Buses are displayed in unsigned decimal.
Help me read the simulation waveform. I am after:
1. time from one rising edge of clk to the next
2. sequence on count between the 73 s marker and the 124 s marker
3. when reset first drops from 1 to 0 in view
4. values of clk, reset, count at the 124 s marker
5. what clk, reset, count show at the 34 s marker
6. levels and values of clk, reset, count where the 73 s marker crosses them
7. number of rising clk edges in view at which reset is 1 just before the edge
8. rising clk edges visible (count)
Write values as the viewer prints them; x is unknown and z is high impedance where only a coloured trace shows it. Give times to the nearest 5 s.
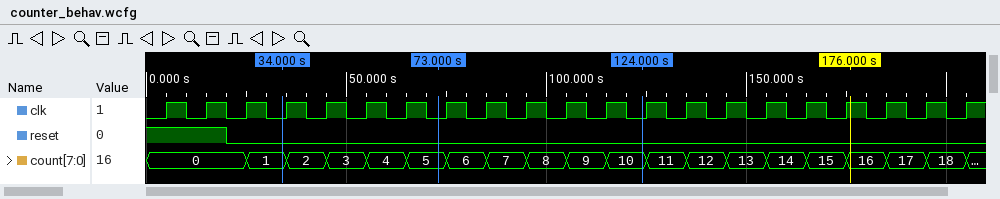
10 s
5, 6, 7, 8, 9, 10
20 s
clk=0, reset=0, count=10
clk=0, reset=0, count=1
clk=0, reset=0, count=5
2
21
